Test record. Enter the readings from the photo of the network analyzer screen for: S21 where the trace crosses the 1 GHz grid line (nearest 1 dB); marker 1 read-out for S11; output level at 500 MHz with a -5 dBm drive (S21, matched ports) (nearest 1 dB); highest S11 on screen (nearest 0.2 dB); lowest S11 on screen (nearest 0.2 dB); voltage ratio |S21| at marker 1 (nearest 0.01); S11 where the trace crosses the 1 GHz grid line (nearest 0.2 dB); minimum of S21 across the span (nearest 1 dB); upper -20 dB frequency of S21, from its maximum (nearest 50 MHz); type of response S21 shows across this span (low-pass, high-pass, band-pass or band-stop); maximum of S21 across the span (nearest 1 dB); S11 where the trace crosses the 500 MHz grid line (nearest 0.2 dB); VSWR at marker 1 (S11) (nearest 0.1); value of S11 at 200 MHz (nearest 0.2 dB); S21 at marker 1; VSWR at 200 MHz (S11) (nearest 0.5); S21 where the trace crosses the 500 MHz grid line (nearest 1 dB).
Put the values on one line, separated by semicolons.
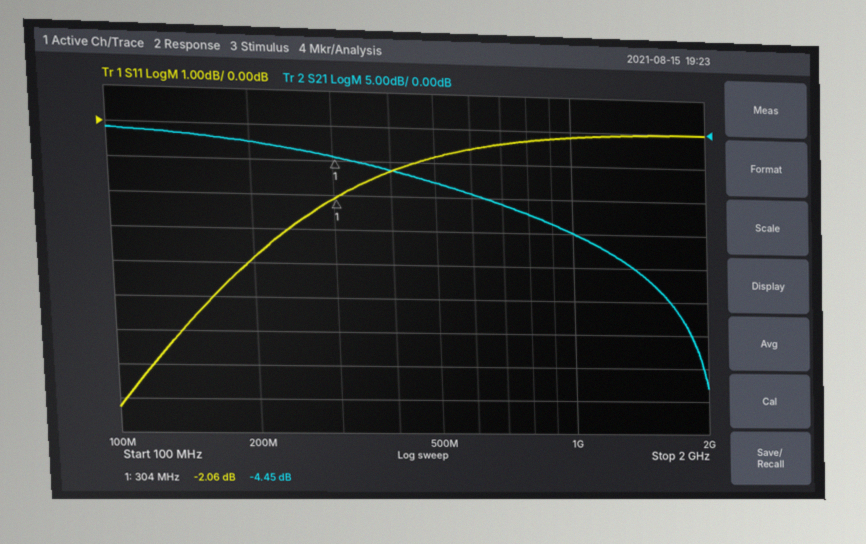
-15 dB; -2.06 dB; -13 dBm; 0.0 dB; -8.2 dB; 0.60; -0.2 dB; -38 dB; 1.40 GHz; low-pass; -1 dB; -0.8 dB; 8.5; -3.8 dB; -4.45 dB; 4.5; -8 dB
